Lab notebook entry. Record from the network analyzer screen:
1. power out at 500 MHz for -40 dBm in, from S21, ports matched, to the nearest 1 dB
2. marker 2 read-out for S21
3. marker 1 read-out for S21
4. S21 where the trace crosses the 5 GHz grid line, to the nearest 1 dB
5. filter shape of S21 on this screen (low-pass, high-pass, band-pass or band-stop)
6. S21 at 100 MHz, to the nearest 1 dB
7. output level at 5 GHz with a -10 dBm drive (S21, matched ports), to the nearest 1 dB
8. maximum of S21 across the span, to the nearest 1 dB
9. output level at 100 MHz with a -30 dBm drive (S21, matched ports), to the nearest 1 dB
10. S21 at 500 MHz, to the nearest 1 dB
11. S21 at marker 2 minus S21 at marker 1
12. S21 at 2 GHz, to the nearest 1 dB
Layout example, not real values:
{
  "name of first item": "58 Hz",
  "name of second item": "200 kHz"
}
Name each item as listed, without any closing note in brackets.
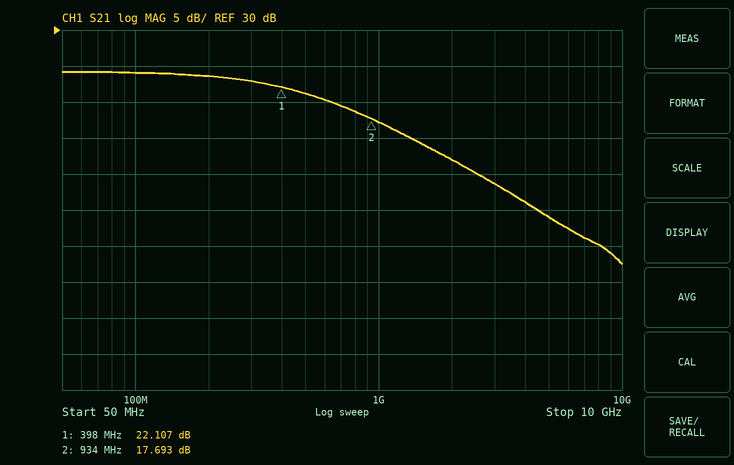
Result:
{
  "power out at 500 MHz for -40 dBm in, from S21, ports matched, to the nearest 1 dB": "-19 dBm",
  "marker 2 read-out for S21": "17.693 dB",
  "marker 1 read-out for S21": "22.107 dB",
  "S21 where the trace crosses the 5 GHz grid line, to the nearest 1 dB": "4 dB",
  "filter shape of S21 on this screen": "low-pass",
  "S21 at 100 MHz, to the nearest 1 dB": "24 dB",
  "output level at 5 GHz with a -10 dBm drive (S21, matched ports), to the nearest 1 dB": "-6 dBm",
  "maximum of S21 across the span, to the nearest 1 dB": "24 dB",
  "output level at 100 MHz with a -30 dBm drive (S21, matched ports), to the nearest 1 dB": "-6 dBm",
  "S21 at 500 MHz, to the nearest 1 dB": "21 dB",
  "S21 at marker 2 minus S21 at marker 1": "-4.414 dB",
  "S21 at 2 GHz, to the nearest 1 dB": "12 dB"
}
